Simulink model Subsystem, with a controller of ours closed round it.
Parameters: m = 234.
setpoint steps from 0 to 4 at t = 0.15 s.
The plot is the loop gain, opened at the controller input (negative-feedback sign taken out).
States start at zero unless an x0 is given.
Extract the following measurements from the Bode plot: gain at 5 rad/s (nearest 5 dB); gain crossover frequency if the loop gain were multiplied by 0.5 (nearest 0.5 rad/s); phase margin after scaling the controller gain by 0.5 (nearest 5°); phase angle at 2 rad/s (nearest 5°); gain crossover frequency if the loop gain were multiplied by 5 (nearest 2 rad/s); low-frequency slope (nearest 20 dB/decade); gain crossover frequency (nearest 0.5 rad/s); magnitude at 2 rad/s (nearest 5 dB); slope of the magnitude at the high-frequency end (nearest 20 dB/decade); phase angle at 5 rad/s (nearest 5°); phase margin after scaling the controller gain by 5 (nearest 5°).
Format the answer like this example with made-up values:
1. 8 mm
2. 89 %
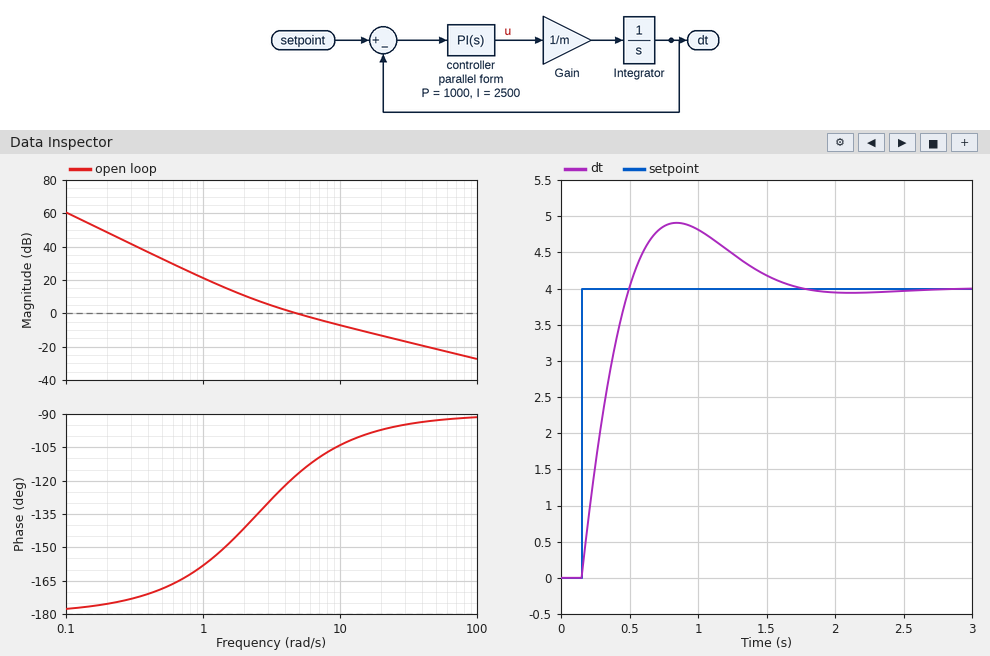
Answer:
1. 0 dB
2. 3.0 rad/s
3. 50°
4. -140°
5. 22 rad/s
6. -40 dB/decade
7. 5.0 rad/s
8. 10 dB
9. -20 dB/decade
10. -115°
11. 85°
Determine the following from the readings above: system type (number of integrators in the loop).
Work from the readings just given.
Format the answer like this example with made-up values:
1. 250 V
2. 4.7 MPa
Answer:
1. 2
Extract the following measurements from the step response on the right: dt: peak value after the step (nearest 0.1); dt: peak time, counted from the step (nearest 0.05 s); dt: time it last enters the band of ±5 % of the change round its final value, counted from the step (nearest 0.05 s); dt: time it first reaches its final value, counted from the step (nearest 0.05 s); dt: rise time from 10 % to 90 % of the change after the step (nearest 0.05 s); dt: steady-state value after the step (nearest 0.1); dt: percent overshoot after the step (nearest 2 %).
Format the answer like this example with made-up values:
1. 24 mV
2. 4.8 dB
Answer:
1. 4.9
2. 0.70 s
3. 1.35 s
4. 0.35 s
5. 0.25 s
6. 4.0
7. 22 %
